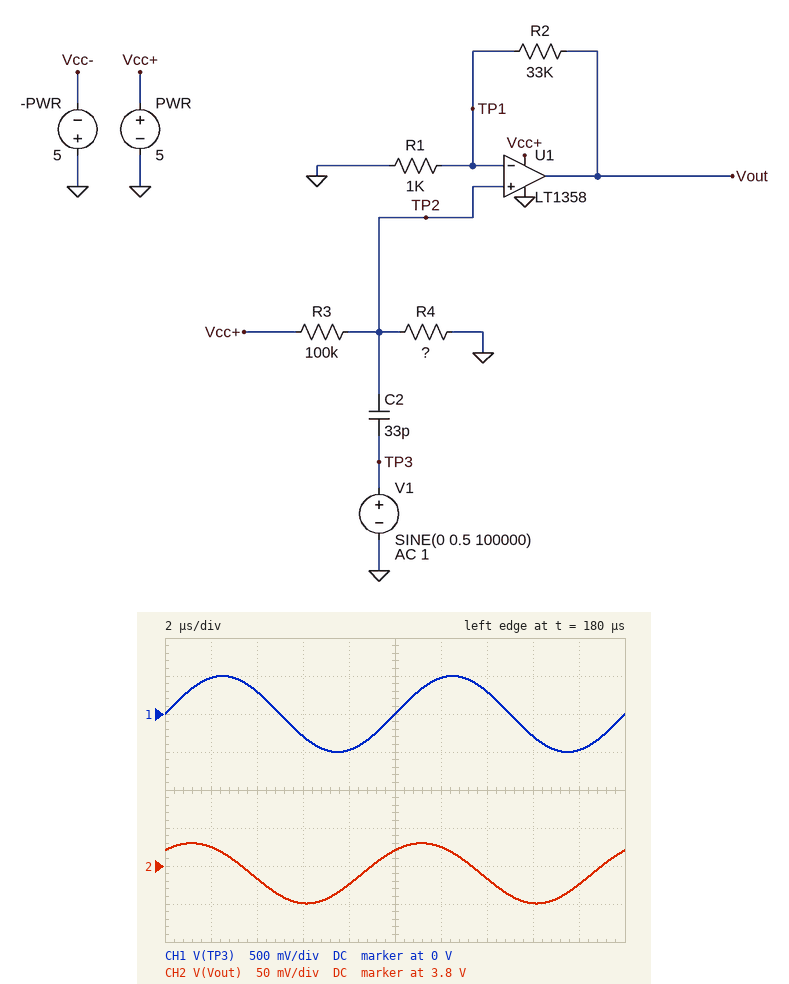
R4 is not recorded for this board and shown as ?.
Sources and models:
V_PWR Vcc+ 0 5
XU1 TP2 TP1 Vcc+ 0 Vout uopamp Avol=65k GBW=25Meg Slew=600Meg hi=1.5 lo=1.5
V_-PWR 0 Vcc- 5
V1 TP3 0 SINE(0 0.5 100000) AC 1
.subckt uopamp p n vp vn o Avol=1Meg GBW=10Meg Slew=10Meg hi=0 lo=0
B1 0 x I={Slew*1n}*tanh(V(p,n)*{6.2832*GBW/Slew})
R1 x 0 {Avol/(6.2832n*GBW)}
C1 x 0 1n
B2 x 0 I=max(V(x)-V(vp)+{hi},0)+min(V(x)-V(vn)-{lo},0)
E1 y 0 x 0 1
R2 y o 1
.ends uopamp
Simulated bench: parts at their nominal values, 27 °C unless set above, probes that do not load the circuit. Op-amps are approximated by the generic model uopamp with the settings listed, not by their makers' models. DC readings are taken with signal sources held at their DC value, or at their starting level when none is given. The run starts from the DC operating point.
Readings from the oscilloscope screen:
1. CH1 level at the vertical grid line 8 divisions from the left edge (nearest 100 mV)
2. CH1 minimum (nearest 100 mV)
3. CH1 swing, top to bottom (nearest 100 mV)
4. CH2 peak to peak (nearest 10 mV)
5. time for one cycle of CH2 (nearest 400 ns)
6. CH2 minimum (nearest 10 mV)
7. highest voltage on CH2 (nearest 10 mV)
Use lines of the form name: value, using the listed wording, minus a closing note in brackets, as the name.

CH1 level at the vertical grid line 8 divisions from the left edge: -300 mV
CH1 minimum: -500 mV
CH1 swing, top to bottom: 1.0 V
CH2 peak to peak: 80 mV
time for one cycle of CH2: 10.0 µs
CH2 minimum: 3.75 V
highest voltage on CH2: 3.83 V
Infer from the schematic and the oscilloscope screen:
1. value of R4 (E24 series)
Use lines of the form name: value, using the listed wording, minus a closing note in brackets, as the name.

value of R4: 75 kΩ
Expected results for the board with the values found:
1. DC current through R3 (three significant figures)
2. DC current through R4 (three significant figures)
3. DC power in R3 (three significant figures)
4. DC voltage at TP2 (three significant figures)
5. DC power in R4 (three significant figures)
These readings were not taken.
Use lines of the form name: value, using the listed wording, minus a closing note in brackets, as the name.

DC current through R3: 28.6 µA
DC current through R4: 28.6 µA
DC power in R3: 81.6 µW
DC voltage at TP2: 2.14 V
DC power in R4: 61.2 µW
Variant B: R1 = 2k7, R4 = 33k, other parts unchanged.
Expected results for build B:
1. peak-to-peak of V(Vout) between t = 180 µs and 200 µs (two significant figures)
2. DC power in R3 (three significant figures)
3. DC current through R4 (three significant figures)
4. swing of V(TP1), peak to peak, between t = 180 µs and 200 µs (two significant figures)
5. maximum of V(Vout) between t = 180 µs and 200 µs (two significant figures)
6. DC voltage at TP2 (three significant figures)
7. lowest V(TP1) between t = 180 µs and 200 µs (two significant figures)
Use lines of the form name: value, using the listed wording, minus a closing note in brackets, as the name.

peak-to-peak of V(Vout) between t = 180 µs and 200 µs: 67 mV
DC power in R3: 141 µW
DC current through R4: 37.6 µA
swing of V(TP1), peak to peak, between t = 180 µs and 200 µs: 5.0 mV
maximum of V(Vout) between t = 180 µs and 200 µs: 3.7 V
DC voltage at TP2: 1.24 V
lowest V(TP1) between t = 180 µs and 200 µs: 270 mV
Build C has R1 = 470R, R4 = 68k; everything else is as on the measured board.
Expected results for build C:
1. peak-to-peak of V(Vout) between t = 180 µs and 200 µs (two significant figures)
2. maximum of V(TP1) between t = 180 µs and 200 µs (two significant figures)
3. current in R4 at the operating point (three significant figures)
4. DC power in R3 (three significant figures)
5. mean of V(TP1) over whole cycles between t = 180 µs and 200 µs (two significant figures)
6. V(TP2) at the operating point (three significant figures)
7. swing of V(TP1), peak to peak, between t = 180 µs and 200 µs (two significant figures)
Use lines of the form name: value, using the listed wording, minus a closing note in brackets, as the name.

peak-to-peak of V(Vout) between t = 180 µs and 200 µs: 78 mV
maximum of V(TP1) between t = 180 µs and 200 µs: 54 mV
current in R4 at the operating point: 29.8 µA
DC power in R3: 88.6 µW
mean of V(TP1) over whole cycles between t = 180 µs and 200 µs: 53 mV
V(TP2) at the operating point: 2.02 V
swing of V(TP1), peak to peak, between t = 180 µs and 200 µs: 1.1 mV
